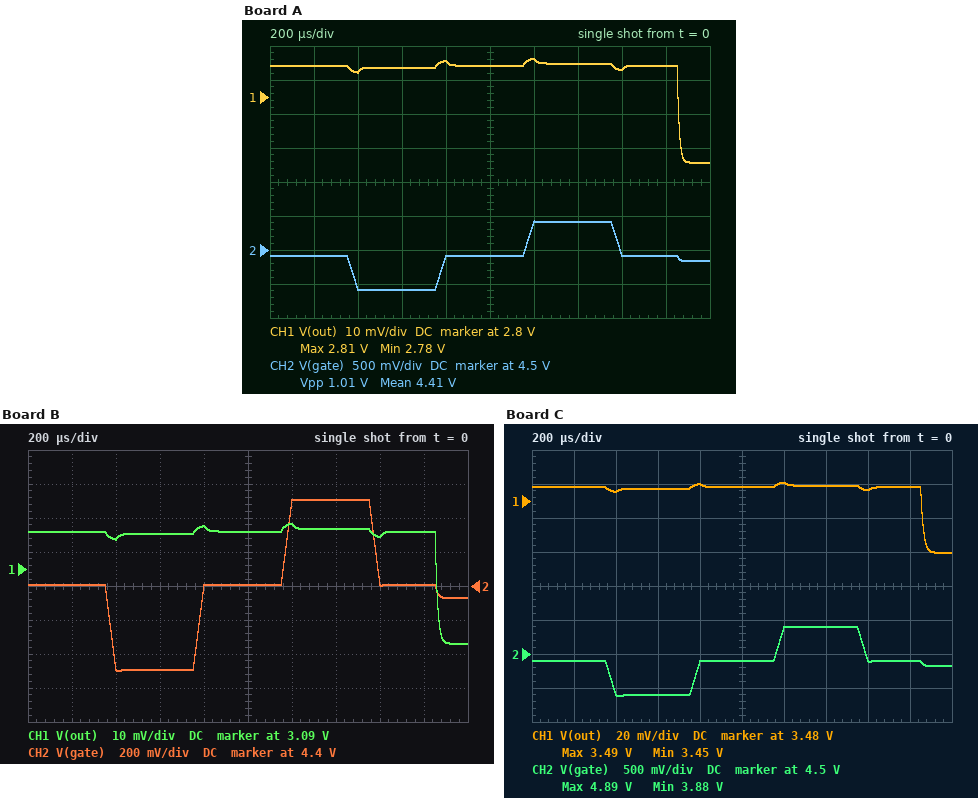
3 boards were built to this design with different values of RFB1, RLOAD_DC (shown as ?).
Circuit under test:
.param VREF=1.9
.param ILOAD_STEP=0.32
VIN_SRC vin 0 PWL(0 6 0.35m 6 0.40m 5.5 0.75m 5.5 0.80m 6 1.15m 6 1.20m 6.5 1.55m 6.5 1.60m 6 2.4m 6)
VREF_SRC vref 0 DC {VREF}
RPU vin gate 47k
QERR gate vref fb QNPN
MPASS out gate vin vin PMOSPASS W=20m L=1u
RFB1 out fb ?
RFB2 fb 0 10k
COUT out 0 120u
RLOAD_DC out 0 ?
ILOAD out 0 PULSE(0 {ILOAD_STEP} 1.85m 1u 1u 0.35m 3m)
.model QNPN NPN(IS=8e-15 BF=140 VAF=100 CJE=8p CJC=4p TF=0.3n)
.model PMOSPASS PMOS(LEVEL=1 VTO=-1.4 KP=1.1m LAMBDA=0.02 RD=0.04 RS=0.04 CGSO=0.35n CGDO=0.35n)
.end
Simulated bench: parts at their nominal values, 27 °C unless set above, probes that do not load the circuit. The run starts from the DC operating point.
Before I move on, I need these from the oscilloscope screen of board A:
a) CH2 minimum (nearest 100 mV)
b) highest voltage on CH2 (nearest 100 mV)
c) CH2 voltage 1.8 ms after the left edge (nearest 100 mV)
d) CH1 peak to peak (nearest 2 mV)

3.9 V
4.9 V
4.4 V
30 mV
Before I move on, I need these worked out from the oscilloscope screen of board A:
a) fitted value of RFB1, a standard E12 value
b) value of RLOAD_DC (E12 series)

15 kΩ
8.2 Ω
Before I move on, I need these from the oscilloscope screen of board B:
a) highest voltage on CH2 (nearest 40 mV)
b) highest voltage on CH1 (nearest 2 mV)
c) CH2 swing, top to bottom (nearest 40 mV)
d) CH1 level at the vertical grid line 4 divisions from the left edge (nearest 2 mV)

4.92 V
3.104 V
1.00 V
3.102 V
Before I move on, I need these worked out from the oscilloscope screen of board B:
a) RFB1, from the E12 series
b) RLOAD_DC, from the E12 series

18 kΩ
8.2 Ω
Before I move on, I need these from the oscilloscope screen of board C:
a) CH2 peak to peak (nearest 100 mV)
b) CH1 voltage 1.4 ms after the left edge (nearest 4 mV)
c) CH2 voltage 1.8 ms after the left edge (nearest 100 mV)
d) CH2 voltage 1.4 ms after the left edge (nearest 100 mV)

1.0 V
3.488 V
4.4 V
4.9 V
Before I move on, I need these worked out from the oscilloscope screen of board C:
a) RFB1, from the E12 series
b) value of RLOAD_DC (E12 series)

22 kΩ
8.2 Ω
